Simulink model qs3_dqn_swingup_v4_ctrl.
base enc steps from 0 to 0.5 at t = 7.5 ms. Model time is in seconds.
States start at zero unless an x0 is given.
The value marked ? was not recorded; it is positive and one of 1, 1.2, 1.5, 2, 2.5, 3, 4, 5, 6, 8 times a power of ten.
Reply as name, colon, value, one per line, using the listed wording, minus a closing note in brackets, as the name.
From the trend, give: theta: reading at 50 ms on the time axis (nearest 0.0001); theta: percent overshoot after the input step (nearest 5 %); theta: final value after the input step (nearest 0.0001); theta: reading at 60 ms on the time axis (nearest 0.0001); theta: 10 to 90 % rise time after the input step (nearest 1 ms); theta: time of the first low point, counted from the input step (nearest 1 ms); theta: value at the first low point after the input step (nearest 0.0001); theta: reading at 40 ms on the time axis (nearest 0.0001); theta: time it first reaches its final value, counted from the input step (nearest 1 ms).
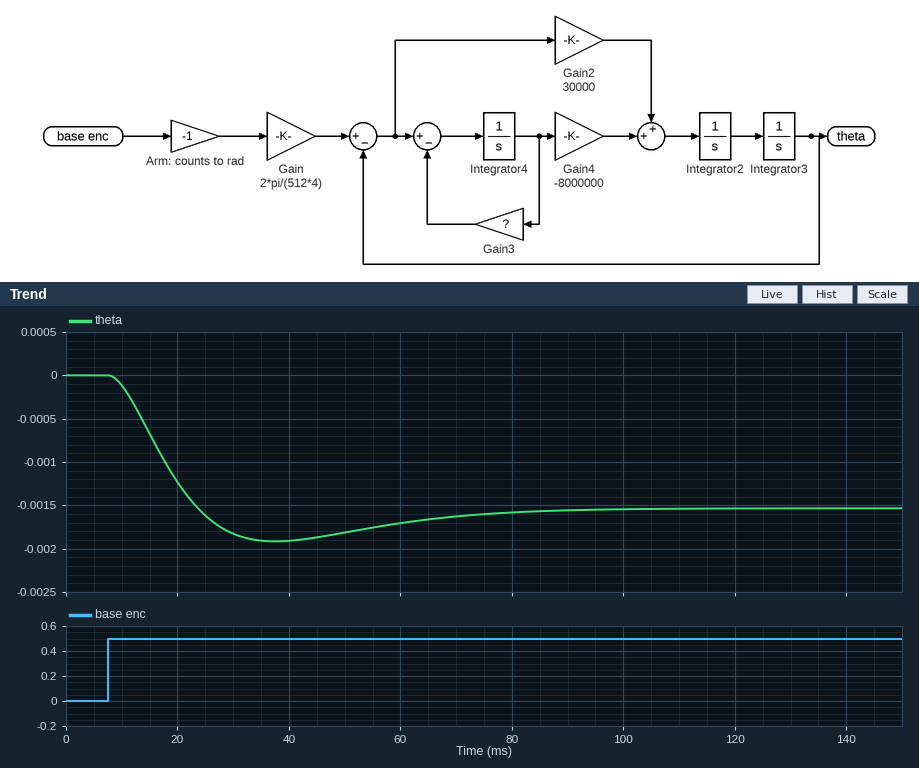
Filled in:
theta: reading at 50 ms on the time axis: -0.0018
theta: percent overshoot after the input step: 25 %
theta: final value after the input step: -0.0015
theta: reading at 60 ms on the time axis: -0.0017
theta: 10 to 90 % rise time after the input step: 11 ms
theta: time of the first low point, counted from the input step: 30 ms
theta: value at the first low point after the input step: -0.0019
theta: reading at 40 ms on the time axis: -0.0019
theta: time it first reaches its final value, counted from the input step: 16 ms
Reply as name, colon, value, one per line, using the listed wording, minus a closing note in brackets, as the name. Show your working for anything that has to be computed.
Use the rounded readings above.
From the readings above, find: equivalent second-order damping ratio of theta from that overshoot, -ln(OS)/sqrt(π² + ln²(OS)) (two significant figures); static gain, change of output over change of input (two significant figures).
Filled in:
equivalent second-order damping ratio of theta from that overshoot, -ln(OS)/sqrt(π² + ln²(OS)): ln(0.25) = -1.386; 1.386 / sqrt(9.870 + 1.922) = 0.40
static gain, change of output over change of input: (-0.0015 - 0) / (0.5 - 0) = -0.0030
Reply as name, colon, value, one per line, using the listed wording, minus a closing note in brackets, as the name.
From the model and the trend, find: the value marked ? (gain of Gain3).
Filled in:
the value marked ?: 300
